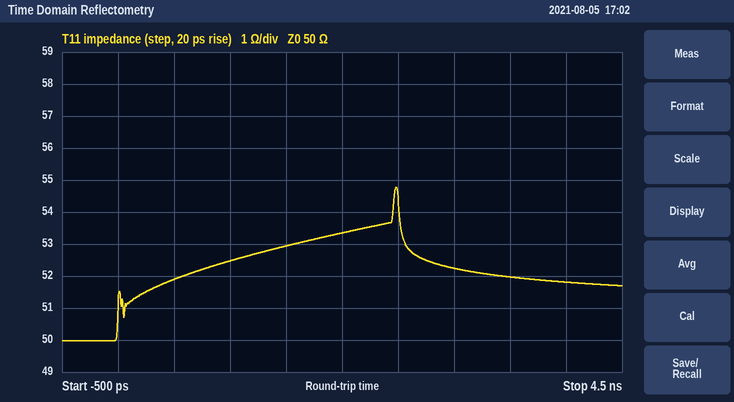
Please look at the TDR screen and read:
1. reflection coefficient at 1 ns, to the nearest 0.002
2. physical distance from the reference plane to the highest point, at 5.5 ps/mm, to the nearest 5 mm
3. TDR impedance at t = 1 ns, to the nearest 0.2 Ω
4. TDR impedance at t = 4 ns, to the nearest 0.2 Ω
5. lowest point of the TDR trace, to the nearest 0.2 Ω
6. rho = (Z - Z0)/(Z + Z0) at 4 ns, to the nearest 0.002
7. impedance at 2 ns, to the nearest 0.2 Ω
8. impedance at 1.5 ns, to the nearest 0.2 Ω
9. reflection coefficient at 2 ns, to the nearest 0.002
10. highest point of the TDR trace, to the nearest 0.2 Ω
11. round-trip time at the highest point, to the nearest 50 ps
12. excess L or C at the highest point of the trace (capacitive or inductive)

+0.024
225 mm
52.4 Ω
51.8 Ω
50.0 Ω
+0.018
53.4 Ω
53.0 Ω
+0.032
54.8 Ω
2.50 ns
inductive
